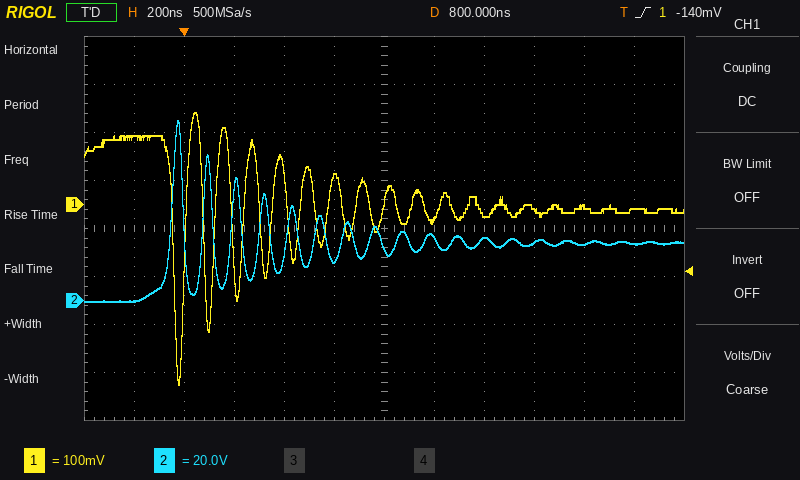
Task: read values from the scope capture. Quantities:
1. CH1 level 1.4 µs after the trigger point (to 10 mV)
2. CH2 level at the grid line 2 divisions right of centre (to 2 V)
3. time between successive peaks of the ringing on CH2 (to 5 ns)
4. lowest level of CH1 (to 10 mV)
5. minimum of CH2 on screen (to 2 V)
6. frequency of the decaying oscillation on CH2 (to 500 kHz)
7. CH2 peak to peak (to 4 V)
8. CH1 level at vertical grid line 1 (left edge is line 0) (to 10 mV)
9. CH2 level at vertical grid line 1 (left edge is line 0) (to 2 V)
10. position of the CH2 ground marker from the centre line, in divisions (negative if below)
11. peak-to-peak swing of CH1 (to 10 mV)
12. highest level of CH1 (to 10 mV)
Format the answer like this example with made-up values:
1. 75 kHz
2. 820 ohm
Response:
1. -10 mV
2. 26 V
3. 110 ns
4. -380 mV
5. 0 V
6. 9.0 MHz
7. 76 V
8. 140 mV
9. 0 V
10. -1.5 div
11. 570 mV
12. 190 mV
